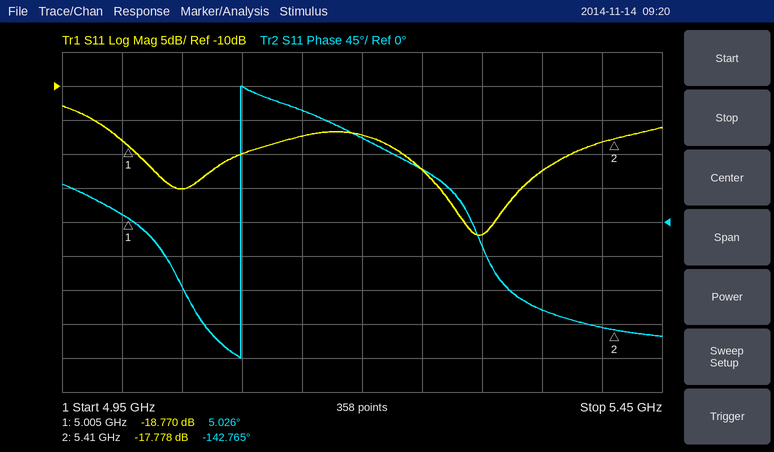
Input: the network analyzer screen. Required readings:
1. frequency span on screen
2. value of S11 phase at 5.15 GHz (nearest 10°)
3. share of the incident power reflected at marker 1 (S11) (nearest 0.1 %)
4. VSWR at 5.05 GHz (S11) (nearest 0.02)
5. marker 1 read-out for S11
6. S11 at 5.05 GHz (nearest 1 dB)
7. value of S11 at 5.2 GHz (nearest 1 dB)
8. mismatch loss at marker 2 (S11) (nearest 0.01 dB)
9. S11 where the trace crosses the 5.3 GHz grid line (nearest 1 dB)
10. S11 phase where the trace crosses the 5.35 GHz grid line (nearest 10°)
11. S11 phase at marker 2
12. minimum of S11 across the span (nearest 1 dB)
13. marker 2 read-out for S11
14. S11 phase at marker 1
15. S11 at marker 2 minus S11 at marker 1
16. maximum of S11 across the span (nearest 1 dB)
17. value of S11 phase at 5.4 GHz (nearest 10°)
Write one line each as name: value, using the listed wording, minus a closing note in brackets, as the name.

frequency span on screen: 500 MHz
value of S11 phase at 5.15 GHz: 150°
share of the incident power reflected at marker 1 (S11): 1.3 %
VSWR at 5.05 GHz (S11): 1.12
marker 1 read-out for S11: -18.770 dB
S11 at 5.05 GHz: -25 dB
value of S11 at 5.2 GHz: -17 dB
mismatch loss at marker 2 (S11): 0.07 dB
S11 where the trace crosses the 5.3 GHz grid line: -32 dB
S11 phase where the trace crosses the 5.35 GHz grid line: -120°
S11 phase at marker 2: -142.765°
minimum of S11 across the span: -32 dB
marker 2 read-out for S11: -17.778 dB
S11 phase at marker 1: 5.026°
S11 at marker 2 minus S11 at marker 1: 0.992 dB
maximum of S11 across the span: -13 dB
value of S11 phase at 5.4 GHz: -140°
